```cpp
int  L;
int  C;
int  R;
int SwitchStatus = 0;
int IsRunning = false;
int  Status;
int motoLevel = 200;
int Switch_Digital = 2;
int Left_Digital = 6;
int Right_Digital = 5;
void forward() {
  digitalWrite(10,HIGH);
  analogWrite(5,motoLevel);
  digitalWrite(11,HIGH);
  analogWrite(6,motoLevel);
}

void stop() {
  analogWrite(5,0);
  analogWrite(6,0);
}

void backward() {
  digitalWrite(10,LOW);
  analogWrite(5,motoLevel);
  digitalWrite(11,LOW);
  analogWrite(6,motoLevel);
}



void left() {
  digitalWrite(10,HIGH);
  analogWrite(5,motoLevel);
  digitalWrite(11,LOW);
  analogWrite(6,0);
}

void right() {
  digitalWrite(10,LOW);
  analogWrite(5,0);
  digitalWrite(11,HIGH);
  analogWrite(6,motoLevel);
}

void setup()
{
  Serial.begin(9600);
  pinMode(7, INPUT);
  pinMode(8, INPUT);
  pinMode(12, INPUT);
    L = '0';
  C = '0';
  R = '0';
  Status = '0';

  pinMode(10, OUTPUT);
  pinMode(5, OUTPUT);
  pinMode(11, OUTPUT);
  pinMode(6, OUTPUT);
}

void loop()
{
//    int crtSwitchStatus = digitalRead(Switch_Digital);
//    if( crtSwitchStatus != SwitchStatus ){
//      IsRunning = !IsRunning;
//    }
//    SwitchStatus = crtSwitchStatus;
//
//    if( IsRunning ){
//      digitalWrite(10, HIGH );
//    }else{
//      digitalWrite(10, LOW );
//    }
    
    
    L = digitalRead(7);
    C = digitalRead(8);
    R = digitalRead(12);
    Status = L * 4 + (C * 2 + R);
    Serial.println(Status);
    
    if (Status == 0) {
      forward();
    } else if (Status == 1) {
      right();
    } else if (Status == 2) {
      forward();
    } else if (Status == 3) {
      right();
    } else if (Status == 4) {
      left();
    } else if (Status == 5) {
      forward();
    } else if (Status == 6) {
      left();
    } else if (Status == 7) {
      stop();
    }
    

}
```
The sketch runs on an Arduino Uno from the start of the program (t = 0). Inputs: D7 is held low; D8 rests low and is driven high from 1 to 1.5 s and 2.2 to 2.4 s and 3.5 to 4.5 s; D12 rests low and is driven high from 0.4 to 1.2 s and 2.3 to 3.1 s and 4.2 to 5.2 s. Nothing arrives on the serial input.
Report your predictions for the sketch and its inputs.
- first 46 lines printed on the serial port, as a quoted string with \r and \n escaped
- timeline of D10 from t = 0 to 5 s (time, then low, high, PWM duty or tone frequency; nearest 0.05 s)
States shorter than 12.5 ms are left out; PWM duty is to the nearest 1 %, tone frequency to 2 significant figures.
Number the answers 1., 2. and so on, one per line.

1. "0\r\n0\r\n0\r\n0\r\n0\r\n0\r\n0\r\n0\r\n0\r\n0\r\n0\r\n0\r\n0\r\n0\r\n0\r\n0\r\n0\r\n0\r\n0\r\n0\r\n0\r\n0\r\n0\r\n0\r\n0\r\n0\r\n0\r\n0\r\n0\r\n0\r\n0\r\n0\r\n0\r\n0\r\n0\r\n0\r\n0\r\n0\r\n0\r\n0\r\n0\r\n0\r\n0\r\n0\r\n0\r\n0\r\n"
2. 0 s high; 0.4 s low; 1.2 s high; 2.3 s low; 3.1 s high; 4.2 s low
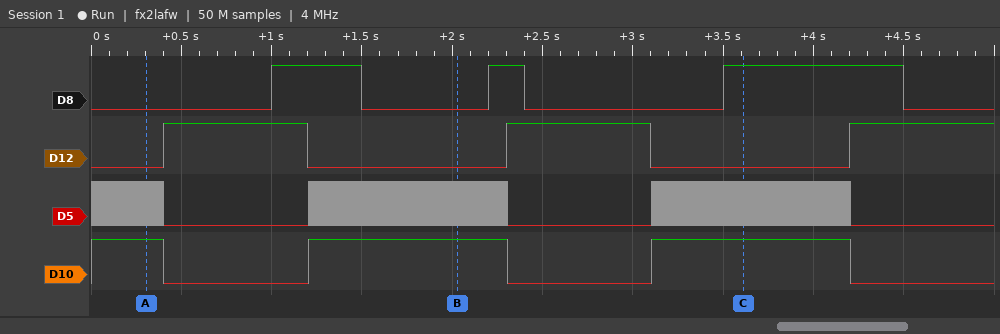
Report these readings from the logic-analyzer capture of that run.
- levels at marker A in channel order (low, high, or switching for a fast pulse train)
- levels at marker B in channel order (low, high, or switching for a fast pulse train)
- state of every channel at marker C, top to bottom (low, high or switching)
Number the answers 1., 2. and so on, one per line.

1. D8 low, D12 low, D5 switching, D10 high
2. D8 low, D12 low, D5 switching, D10 high
3. D8 high, D12 low, D5 switching, D10 high
